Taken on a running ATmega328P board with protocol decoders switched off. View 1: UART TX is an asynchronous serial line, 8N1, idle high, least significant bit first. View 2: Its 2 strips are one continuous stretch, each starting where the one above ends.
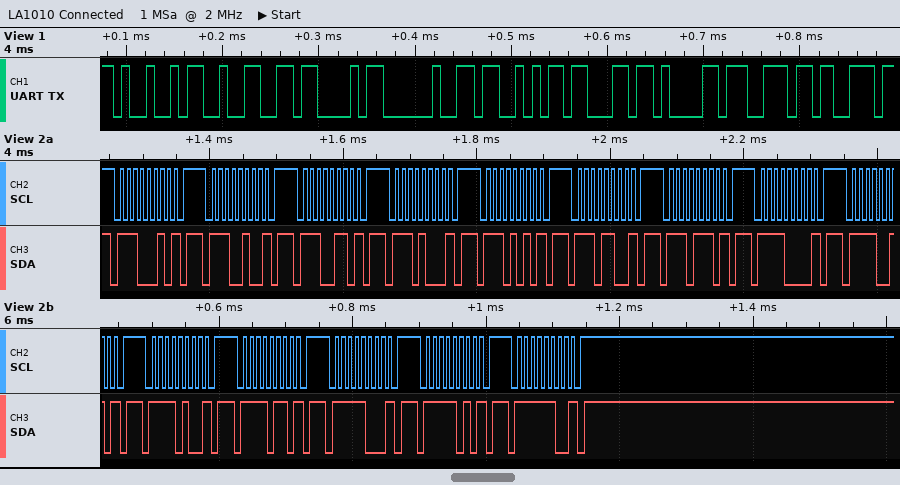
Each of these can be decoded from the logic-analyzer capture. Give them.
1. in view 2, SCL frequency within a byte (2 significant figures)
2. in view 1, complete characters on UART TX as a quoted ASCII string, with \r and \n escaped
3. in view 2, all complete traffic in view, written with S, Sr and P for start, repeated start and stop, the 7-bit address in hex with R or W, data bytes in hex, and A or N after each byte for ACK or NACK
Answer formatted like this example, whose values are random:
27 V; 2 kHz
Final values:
100 kHz; "I2C Scan"; S 71W N P S 72W N P S 73W N P S 74W N P S 75W N P S 76W N P S 77W N P S 78W N P S 79W N P S 7AW N P S 7BW N P S 7CW N P S 7DW N P S 7EW N P
